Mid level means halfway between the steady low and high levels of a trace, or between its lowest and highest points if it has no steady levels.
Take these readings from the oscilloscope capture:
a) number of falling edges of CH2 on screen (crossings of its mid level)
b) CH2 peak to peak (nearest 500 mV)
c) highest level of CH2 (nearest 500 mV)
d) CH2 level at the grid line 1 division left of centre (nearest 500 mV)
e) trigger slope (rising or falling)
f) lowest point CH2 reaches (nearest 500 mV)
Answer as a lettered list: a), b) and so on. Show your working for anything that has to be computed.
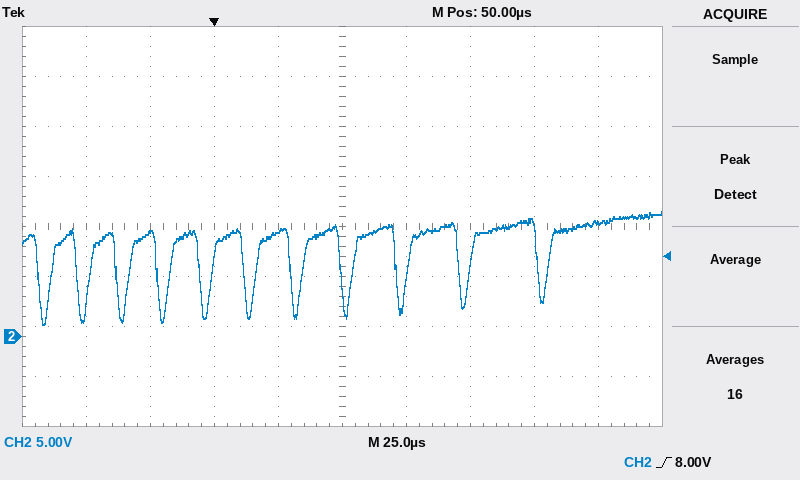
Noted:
a) 11
b) 12.5 V − (1.0 V) = 11.5 V
c) 12.5 V
d) 10.5 V
e) rising
f) 1.0 V
